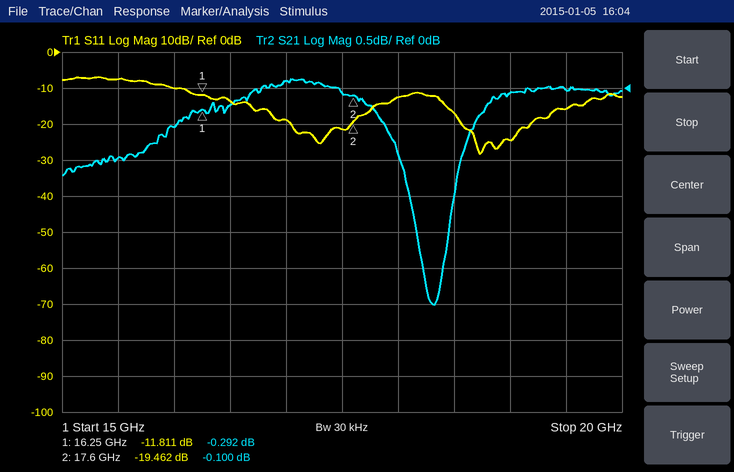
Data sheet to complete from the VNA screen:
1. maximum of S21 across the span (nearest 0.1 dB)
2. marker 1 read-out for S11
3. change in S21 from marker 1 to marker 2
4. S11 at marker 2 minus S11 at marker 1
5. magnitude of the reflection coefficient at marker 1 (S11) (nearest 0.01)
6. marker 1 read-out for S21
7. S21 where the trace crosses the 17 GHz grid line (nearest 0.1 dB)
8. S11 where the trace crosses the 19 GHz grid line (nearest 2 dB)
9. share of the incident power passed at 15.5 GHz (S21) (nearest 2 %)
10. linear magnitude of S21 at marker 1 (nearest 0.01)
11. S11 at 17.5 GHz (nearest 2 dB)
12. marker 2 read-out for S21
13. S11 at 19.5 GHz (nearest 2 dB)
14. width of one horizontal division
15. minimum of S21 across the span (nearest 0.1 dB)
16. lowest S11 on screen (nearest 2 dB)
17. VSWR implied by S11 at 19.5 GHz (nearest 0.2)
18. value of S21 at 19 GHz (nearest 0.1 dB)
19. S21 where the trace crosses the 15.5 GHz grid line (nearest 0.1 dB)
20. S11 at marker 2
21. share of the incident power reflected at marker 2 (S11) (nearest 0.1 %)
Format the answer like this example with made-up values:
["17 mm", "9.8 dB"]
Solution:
["0.1 dB", "-11.811 dB", "0.192 dB", "-7.651 dB", "0.26", "-0.292 dB", "0.1 dB", "-24 dB", "80 %", "0.97", "-22 dB", "-0.100 dB", "-16 dB", "500 MHz", "-3.0 dB", "-28 dB", "1.4", "-0.1 dB", "-1.0 dB", "-19.462 dB", "1.1 %"]
